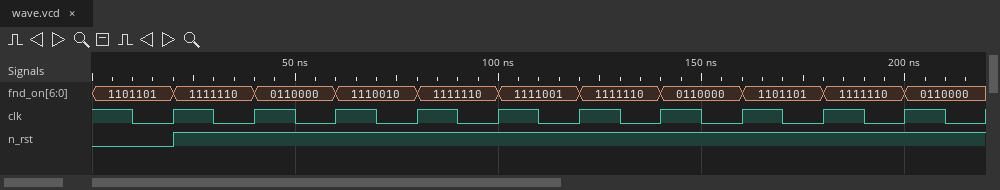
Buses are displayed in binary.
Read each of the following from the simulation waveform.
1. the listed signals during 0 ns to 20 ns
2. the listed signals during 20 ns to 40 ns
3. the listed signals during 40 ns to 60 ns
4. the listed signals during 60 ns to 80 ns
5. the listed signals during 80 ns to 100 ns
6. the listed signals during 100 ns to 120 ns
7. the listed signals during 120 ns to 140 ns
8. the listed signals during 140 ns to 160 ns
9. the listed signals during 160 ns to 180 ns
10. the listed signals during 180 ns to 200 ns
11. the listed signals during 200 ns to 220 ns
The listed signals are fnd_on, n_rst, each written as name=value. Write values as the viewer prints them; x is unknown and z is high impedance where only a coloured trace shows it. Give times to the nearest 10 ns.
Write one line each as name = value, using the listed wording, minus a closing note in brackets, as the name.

the listed signals during 0 ns to 20 ns = fnd_on=1101101, n_rst=0
the listed signals during 20 ns to 40 ns = fnd_on=1111110, n_rst=1
the listed signals during 40 ns to 60 ns = fnd_on=0110000, n_rst=1
the listed signals during 60 ns to 80 ns = fnd_on=1110010, n_rst=1
the listed signals during 80 ns to 100 ns = fnd_on=1111110, n_rst=1
the listed signals during 100 ns to 120 ns = fnd_on=1111001, n_rst=1
the listed signals during 120 ns to 140 ns = fnd_on=1111110, n_rst=1
the listed signals during 140 ns to 160 ns = fnd_on=0110000, n_rst=1
the listed signals during 160 ns to 180 ns = fnd_on=1101101, n_rst=1
the listed signals during 180 ns to 200 ns = fnd_on=1111110, n_rst=1
the listed signals during 200 ns to 220 ns = fnd_on=0110000, n_rst=1
